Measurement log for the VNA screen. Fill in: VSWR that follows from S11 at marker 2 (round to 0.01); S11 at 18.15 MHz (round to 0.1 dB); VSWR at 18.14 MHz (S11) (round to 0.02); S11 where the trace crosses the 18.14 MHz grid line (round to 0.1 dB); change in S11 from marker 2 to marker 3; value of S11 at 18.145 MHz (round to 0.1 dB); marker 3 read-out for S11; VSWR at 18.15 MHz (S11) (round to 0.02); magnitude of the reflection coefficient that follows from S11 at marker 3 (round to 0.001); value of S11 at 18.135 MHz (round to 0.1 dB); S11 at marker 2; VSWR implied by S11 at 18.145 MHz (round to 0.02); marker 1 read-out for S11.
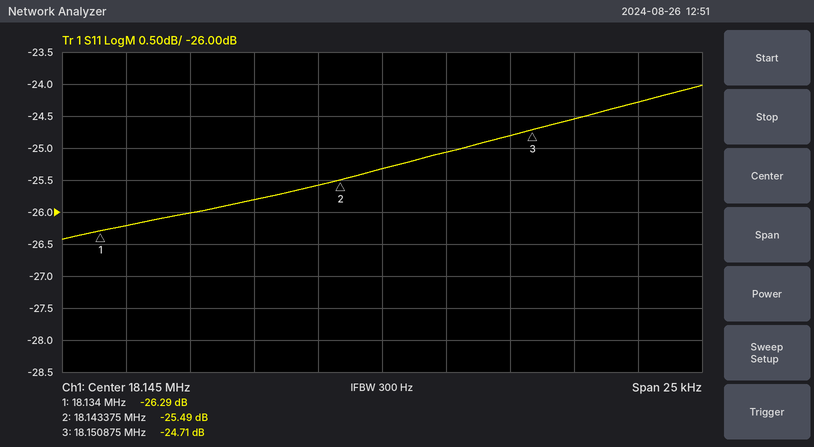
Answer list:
1.11
-24.8 dB
1.10
-25.8 dB
0.78 dB
-25.3 dB
-24.71 dB
1.12
0.058
-26.2 dB
-25.49 dB
1.12
-26.29 dB
